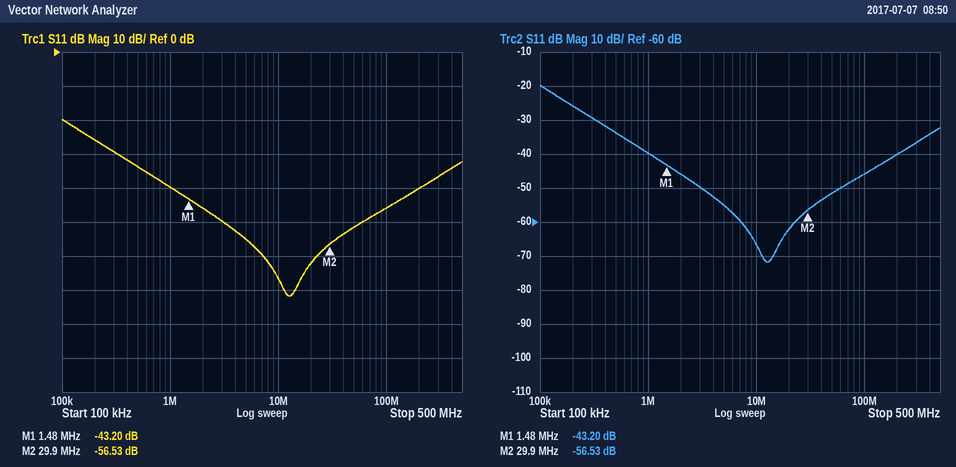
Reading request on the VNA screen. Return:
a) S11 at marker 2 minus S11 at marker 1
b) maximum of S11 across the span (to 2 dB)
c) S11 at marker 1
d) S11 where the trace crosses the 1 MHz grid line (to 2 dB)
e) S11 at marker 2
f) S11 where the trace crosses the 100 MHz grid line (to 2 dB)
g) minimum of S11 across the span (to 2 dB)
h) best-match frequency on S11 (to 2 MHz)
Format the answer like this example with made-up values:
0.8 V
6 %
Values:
-13.33 dB
-20 dB
-43.20 dB
-40 dB
-56.53 dB
-46 dB
-72 dB
12 MHz
